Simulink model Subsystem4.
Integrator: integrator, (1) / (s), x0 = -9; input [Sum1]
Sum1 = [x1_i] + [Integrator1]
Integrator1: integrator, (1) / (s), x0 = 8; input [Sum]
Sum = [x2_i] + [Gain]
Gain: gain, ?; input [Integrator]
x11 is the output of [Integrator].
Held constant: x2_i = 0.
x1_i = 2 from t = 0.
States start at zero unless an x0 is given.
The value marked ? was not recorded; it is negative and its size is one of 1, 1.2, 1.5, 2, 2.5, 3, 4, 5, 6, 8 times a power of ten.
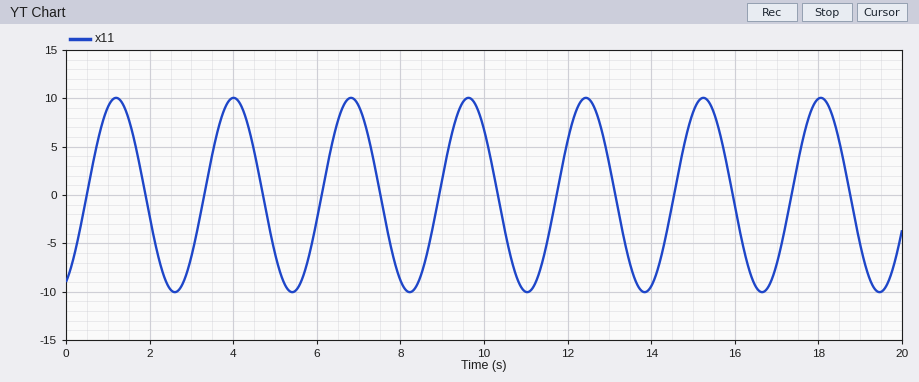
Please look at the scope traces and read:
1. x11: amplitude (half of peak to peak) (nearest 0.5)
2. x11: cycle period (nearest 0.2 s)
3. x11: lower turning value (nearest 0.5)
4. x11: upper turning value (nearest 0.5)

10.0
2.8 s
-10.0
10.0
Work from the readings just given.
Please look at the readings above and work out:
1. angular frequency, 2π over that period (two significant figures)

2.2 rad/s
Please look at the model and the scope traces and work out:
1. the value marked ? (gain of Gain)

-5
